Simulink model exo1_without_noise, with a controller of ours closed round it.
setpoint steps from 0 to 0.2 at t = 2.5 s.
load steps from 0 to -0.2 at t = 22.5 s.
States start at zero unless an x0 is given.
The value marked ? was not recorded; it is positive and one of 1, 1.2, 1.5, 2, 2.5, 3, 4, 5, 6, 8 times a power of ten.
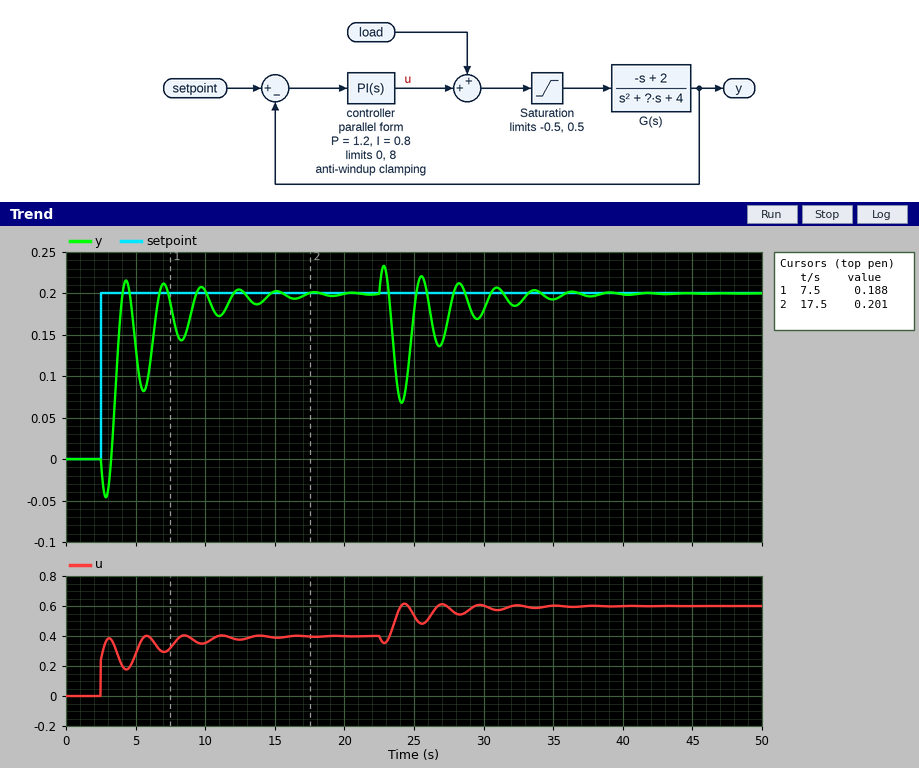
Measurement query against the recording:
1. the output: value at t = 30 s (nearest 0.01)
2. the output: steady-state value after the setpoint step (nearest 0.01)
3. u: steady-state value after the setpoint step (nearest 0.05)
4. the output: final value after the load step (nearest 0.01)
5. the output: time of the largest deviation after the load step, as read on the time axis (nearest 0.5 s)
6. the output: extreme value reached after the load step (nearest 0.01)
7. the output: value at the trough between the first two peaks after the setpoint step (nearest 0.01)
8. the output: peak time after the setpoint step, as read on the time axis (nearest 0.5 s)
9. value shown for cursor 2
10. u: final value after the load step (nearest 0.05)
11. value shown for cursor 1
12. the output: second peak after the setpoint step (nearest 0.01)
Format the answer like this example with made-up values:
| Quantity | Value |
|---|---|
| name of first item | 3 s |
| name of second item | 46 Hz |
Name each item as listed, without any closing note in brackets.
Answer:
| Quantity | Value |
|---|---|
| the output: value at t = 30 s | 0.18 |
| the output: steady-state value after the setpoint step | 0.20 |
| u: steady-state value after the setpoint step | 0.40 |
| the output: final value after the load step | 0.20 |
| the output: time of the largest deviation after the load step, as read on the time axis | 24.0 s |
| the output: extreme value reached after the load step | 0.07 |
| the output: value at the trough between the first two peaks after the setpoint step | 0.08 |
| the output: peak time after the setpoint step, as read on the time axis | 4.5 s |
| value shown for cursor 2 | 0.201 |
| u: final value after the load step | 0.60 |
| value shown for cursor 1 | 0.188 |
| the output: second peak after the setpoint step | 0.21 |
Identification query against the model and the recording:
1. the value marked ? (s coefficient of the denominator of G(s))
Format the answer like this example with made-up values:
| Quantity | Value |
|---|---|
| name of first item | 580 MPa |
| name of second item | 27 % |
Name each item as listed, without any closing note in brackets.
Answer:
| Quantity | Value |
|---|---|
| the value marked ? (s coefficient of the denominator of G(s)) | 2 |
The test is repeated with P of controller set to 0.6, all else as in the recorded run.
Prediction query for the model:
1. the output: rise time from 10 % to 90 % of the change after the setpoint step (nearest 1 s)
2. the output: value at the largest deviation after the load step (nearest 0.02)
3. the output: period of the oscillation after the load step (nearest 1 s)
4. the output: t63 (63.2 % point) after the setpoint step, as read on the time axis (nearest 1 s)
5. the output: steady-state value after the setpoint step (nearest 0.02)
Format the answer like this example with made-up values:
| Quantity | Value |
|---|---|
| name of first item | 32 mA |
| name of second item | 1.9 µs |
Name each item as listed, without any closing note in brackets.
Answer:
| Quantity | Value |
|---|---|
| the output: rise time from 10 % to 90 % of the change after the setpoint step | 4 s |
| the output: value at the largest deviation after the load step | 0.08 |
| the output: period of the oscillation after the load step | 3 s |
| the output: t63 (63.2 % point) after the setpoint step, as read on the time axis | 4 s |
| the output: steady-state value after the setpoint step | 0.20 |
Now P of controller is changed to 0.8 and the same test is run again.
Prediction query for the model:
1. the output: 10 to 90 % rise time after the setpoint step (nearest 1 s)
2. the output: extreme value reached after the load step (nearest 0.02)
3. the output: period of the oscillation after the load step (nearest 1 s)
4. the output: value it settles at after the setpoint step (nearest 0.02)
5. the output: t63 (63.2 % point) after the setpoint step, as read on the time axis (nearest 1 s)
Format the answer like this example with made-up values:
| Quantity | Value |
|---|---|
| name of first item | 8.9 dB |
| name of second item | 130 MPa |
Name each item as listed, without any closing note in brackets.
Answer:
| Quantity | Value |
|---|---|
| the output: 10 to 90 % rise time after the setpoint step | 4 s |
| the output: extreme value reached after the load step | 0.08 |
| the output: period of the oscillation after the load step | 3 s |
| the output: value it settles at after the setpoint step | 0.20 |
| the output: t63 (63.2 % point) after the setpoint step, as read on the time axis | 4 s |
